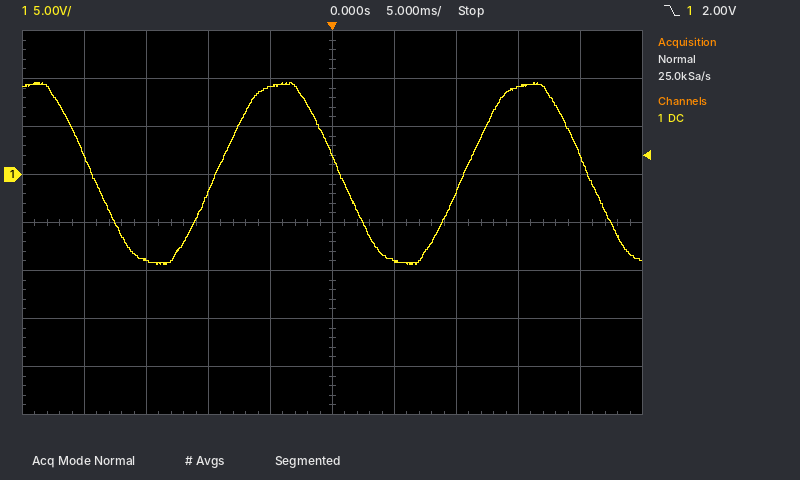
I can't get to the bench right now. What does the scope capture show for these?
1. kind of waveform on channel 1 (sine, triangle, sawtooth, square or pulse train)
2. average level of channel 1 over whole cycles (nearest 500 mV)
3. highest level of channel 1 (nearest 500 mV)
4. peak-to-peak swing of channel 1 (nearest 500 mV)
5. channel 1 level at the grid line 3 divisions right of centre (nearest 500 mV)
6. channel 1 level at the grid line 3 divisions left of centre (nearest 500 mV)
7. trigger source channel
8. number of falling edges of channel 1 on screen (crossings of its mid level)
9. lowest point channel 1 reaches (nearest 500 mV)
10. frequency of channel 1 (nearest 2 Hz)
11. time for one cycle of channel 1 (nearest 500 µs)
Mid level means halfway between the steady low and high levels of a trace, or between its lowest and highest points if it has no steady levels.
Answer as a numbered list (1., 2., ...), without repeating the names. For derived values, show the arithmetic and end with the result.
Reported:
1. sine
2. (9.5 V + (-9.5 V)) / 2 ≈ 0.0 V
3. 9.5 V
4. 9.5 V − (-9.5 V) = 19.0 V
5. 9.0 V
6. -9.0 V
7. channel 1
8. 3
9. -9.5 V
10. 1 / 20.0 ms ≈ 50 Hz
11. 20.0 ms
